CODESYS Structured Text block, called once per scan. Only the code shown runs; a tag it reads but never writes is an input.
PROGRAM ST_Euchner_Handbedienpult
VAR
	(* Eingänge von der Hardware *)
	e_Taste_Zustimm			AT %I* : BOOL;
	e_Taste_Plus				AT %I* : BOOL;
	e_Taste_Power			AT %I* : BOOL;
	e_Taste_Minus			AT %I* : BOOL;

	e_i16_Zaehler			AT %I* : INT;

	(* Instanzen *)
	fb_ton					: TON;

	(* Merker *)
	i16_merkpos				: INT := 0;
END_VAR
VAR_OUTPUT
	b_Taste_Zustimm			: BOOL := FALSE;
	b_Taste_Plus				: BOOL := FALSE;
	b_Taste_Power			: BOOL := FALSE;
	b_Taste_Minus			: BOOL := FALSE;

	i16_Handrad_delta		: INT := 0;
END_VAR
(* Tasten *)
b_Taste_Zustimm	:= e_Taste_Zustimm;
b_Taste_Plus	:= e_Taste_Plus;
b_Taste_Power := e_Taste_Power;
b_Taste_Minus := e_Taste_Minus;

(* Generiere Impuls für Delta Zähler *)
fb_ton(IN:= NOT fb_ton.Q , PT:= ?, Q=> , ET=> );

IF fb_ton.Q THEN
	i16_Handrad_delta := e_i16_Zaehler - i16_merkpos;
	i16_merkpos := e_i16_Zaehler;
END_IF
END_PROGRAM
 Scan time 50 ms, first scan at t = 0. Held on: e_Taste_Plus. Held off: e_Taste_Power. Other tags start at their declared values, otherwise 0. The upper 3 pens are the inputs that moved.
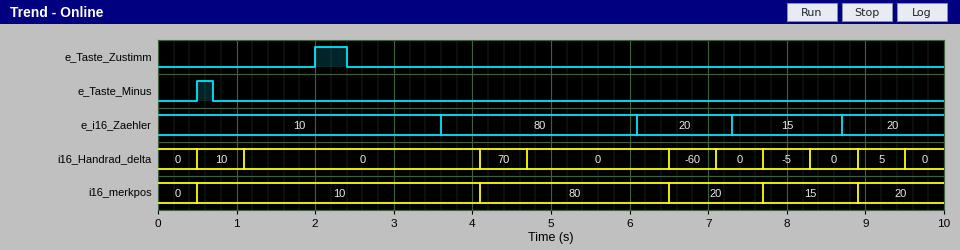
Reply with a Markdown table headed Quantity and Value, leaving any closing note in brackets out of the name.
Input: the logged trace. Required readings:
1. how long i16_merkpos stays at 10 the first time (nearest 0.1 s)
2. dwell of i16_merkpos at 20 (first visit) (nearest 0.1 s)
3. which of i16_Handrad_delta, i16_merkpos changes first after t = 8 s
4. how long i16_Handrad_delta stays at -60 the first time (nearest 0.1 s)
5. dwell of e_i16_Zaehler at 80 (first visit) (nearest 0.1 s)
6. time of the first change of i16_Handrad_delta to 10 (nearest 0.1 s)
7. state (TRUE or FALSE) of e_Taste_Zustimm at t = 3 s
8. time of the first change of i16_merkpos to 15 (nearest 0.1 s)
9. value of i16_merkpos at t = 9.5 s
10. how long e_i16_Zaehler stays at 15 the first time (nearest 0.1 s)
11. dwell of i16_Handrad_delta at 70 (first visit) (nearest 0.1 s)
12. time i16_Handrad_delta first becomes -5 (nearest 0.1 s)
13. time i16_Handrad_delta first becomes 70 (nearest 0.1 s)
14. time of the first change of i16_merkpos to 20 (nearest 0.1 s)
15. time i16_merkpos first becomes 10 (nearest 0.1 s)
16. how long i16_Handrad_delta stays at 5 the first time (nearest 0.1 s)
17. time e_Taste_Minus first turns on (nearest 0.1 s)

| Quantity | Value |
|---|---|
| how long i16_merkpos stays at 10 the first time | 3.6 s |
| dwell of i16_merkpos at 20 (first visit) | 1.2 s |
| which of i16_Handrad_delta, i16_merkpos changes first after t = 8 s | i16_Handrad_delta |
| how long i16_Handrad_delta stays at -60 the first time | 0.6 s |
| dwell of e_i16_Zaehler at 80 (first visit) | 2.5 s |
| time of the first change of i16_Handrad_delta to 10 | 0.5 s |
| state (TRUE or FALSE) of e_Taste_Zustimm at t = 3 s | FALSE |
| time of the first change of i16_merkpos to 15 | 7.7 s |
| value of i16_merkpos at t = 9.5 s | 20 |
| how long e_i16_Zaehler stays at 15 the first time | 1.4 s |
| dwell of i16_Handrad_delta at 70 (first visit) | 0.6 s |
| time i16_Handrad_delta first becomes -5 | 7.7 s |
| time i16_Handrad_delta first becomes 70 | 4.1 s |
| time of the first change of i16_merkpos to 20 | 6.5 s |
| time i16_merkpos first becomes 10 | 0.5 s |
| how long i16_Handrad_delta stays at 5 the first time | 0.6 s |
| time e_Taste_Minus first turns on | 0.5 s |
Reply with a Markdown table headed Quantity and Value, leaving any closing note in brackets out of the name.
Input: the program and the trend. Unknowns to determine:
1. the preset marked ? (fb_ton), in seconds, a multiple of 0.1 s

| Quantity | Value |
|---|---|
| the preset marked ? (fb_ton), in seconds, a multiple of 0.1 s | 0.5 s |
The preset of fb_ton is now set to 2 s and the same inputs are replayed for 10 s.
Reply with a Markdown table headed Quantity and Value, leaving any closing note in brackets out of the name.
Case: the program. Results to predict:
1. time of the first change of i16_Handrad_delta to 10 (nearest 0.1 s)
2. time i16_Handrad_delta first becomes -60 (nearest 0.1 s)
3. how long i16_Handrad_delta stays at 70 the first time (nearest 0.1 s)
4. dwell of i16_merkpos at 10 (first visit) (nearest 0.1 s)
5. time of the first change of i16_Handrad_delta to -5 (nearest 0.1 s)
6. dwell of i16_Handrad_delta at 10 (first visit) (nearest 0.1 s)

| Quantity | Value |
|---|---|
| time of the first change of i16_Handrad_delta to 10 | 2.0 s |
| time i16_Handrad_delta first becomes -60 | 6.2 s |
| how long i16_Handrad_delta stays at 70 the first time | 2.1 s |
| dwell of i16_merkpos at 10 (first visit) | 2.1 s |
| time of the first change of i16_Handrad_delta to -5 | 8.3 s |
| dwell of i16_Handrad_delta at 10 (first visit) | 2.1 s |
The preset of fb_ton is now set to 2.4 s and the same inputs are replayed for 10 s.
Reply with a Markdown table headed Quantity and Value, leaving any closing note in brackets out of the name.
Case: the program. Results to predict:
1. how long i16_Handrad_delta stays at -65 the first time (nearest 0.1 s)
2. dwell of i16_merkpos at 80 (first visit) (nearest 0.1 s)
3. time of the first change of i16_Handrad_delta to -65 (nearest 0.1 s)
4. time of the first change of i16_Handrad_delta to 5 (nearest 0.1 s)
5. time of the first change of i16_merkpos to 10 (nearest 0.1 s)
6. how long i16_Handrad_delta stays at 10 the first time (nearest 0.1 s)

| Quantity | Value |
|---|---|
| how long i16_Handrad_delta stays at -65 the first time | 2.5 s |
| dwell of i16_merkpos at 80 (first visit) | 2.5 s |
| time of the first change of i16_Handrad_delta to -65 | 7.4 s |
| time of the first change of i16_Handrad_delta to 5 | 9.9 s |
| time of the first change of i16_merkpos to 10 | 2.4 s |
| how long i16_Handrad_delta stays at 10 the first time | 2.5 s |
